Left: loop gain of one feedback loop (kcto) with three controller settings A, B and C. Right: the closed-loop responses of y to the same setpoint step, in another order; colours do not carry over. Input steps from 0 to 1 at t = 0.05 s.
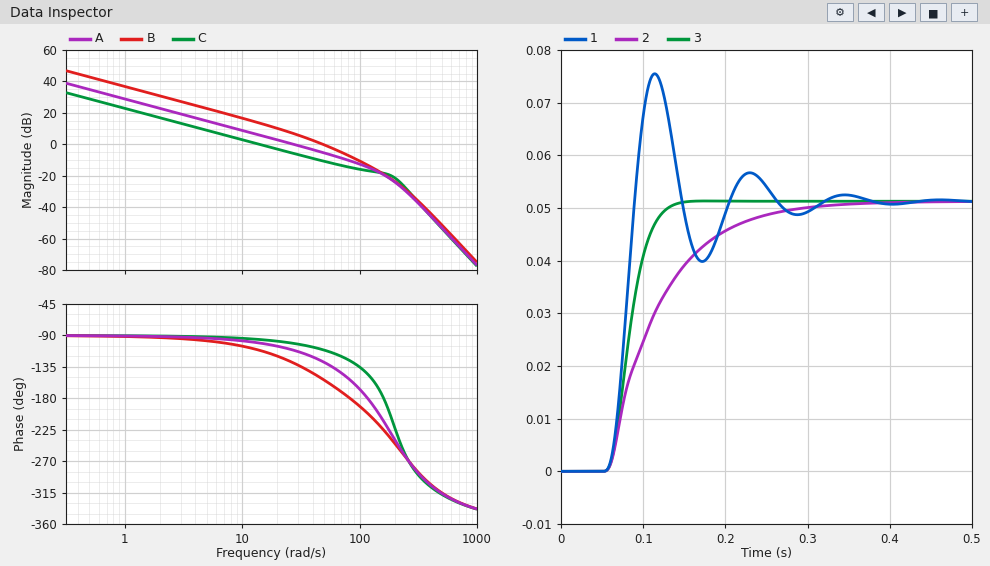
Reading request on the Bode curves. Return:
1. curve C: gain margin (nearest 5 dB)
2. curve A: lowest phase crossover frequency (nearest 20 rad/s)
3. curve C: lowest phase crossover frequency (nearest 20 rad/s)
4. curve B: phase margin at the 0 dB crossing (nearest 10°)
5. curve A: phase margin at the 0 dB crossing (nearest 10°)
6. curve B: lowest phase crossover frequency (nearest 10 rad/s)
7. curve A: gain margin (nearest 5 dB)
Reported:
20 dB
120 rad/s
160 rad/s
30°
70°
80 rad/s
15 dB
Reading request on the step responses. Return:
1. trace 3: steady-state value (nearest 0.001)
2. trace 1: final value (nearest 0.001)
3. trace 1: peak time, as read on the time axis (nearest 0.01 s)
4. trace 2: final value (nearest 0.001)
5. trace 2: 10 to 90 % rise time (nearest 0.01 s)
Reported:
0.051
0.051
0.11 s
0.051
0.14 s
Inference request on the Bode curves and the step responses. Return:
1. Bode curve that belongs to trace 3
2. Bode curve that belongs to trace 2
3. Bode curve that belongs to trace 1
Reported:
A
C
B
